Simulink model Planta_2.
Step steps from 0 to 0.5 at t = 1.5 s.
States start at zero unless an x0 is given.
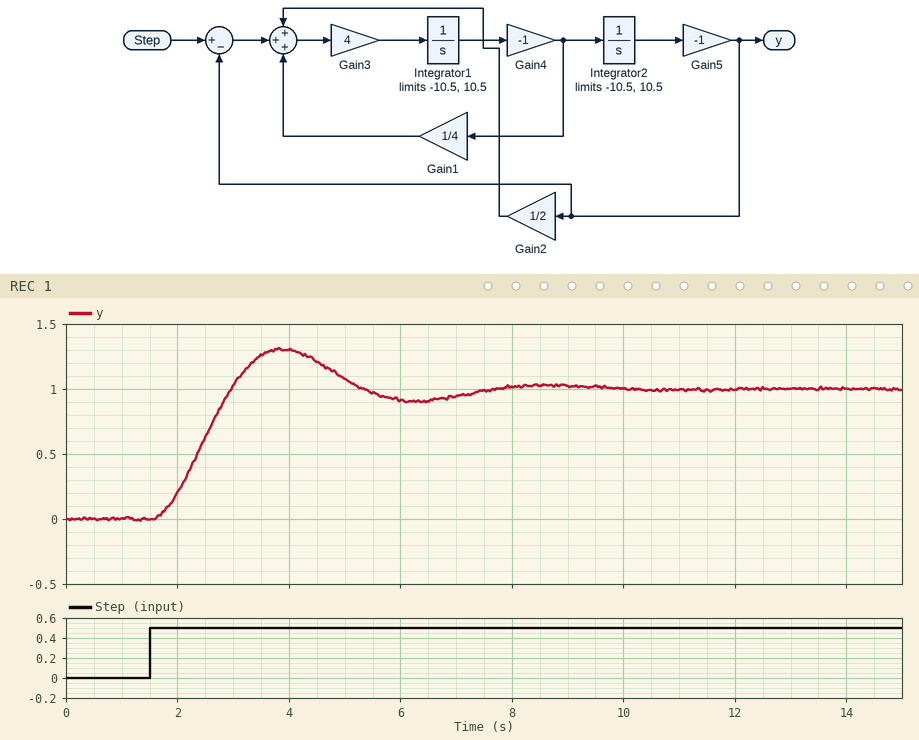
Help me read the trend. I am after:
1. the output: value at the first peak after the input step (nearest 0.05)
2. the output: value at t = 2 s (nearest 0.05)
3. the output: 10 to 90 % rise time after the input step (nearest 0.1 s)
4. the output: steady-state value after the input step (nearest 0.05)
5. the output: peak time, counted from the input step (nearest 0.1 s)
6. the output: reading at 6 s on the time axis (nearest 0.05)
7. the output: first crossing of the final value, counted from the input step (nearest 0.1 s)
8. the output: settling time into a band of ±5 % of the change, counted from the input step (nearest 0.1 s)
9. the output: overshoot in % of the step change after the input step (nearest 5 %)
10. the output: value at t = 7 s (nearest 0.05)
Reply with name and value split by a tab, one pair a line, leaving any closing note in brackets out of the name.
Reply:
the output: value at the first peak after the input step	1.30
the output: value at t = 2 s	0.20
the output: 10 to 90 % rise time after the input step	1.0 s
the output: steady-state value after the input step	1.00
the output: peak time, counted from the input step	2.4 s
the output: reading at 6 s on the time axis	0.90
the output: first crossing of the final value, counted from the input step	1.5 s
the output: settling time into a band of ±5 % of the change, counted from the input step	5.6 s
the output: overshoot in % of the step change after the input step	30 %
the output: value at t = 7 s	0.95
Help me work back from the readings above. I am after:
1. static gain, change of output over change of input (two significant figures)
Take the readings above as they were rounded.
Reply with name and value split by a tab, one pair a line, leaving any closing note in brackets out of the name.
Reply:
static gain, change of output over change of input	2.0
